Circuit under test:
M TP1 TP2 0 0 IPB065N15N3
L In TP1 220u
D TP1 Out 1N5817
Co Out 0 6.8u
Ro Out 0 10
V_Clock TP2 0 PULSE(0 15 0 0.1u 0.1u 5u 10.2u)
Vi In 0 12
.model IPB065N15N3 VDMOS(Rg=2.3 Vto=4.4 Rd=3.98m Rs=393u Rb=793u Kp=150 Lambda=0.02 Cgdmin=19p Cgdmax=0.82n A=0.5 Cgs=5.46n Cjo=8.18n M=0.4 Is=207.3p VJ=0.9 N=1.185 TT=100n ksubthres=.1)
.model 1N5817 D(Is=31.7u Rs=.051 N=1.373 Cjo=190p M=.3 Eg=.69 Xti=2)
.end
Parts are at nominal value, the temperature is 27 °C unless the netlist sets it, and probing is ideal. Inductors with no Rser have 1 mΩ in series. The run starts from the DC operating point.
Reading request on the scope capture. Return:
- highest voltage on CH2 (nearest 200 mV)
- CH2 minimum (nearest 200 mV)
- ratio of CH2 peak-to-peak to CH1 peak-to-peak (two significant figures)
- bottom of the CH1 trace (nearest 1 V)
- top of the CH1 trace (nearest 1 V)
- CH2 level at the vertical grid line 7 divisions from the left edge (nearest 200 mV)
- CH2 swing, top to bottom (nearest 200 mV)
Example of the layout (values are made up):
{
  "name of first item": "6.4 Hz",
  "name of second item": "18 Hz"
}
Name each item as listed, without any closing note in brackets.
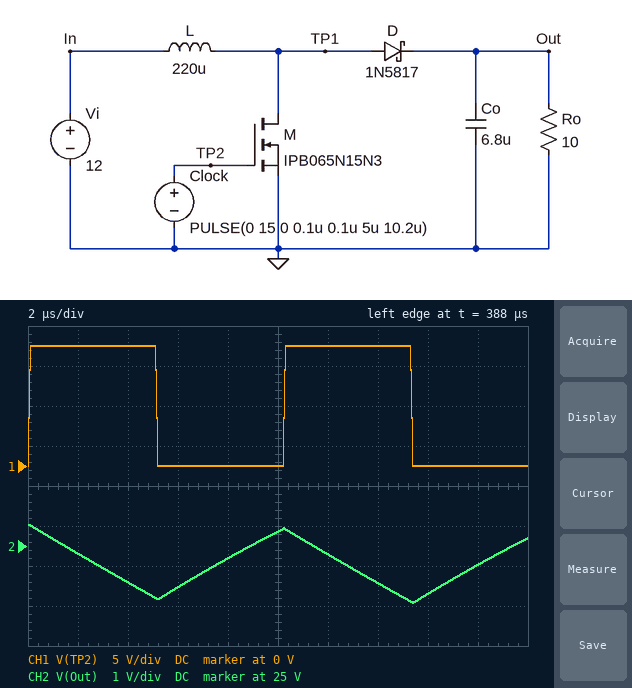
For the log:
{
  "highest voltage on CH2": "25.6 V",
  "CH2 minimum": "23.6 V",
  "ratio of CH2 peak-to-peak to CH1 peak-to-peak": "0.13",
  "bottom of the CH1 trace": "0 V",
  "top of the CH1 trace": "15 V",
  "CH2 level at the vertical grid line 7 divisions from the left edge": "24.0 V",
  "CH2 swing, top to bottom": "2.0 V"
}
